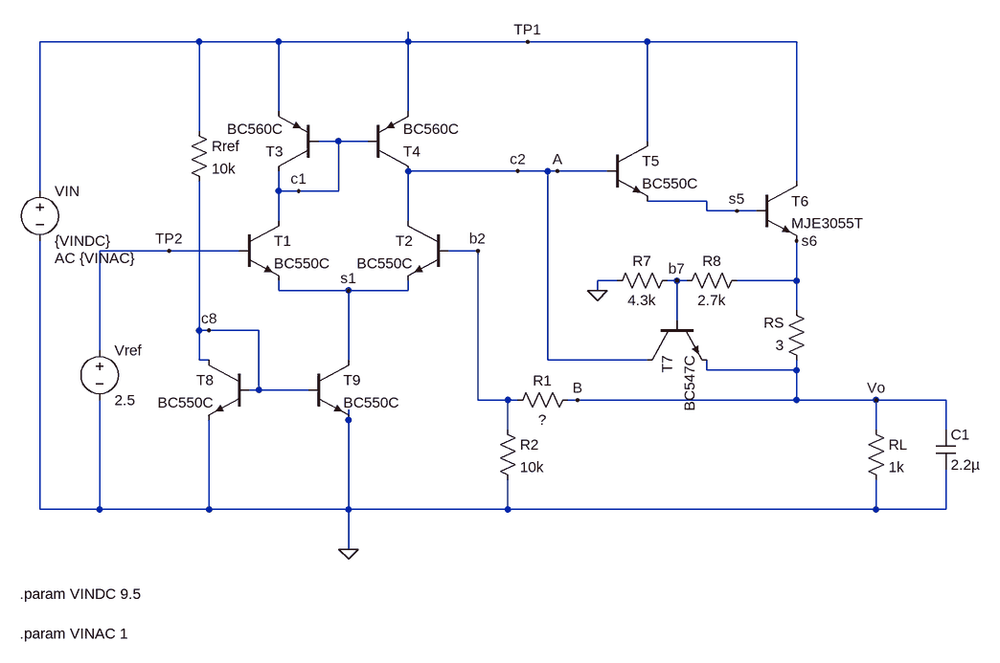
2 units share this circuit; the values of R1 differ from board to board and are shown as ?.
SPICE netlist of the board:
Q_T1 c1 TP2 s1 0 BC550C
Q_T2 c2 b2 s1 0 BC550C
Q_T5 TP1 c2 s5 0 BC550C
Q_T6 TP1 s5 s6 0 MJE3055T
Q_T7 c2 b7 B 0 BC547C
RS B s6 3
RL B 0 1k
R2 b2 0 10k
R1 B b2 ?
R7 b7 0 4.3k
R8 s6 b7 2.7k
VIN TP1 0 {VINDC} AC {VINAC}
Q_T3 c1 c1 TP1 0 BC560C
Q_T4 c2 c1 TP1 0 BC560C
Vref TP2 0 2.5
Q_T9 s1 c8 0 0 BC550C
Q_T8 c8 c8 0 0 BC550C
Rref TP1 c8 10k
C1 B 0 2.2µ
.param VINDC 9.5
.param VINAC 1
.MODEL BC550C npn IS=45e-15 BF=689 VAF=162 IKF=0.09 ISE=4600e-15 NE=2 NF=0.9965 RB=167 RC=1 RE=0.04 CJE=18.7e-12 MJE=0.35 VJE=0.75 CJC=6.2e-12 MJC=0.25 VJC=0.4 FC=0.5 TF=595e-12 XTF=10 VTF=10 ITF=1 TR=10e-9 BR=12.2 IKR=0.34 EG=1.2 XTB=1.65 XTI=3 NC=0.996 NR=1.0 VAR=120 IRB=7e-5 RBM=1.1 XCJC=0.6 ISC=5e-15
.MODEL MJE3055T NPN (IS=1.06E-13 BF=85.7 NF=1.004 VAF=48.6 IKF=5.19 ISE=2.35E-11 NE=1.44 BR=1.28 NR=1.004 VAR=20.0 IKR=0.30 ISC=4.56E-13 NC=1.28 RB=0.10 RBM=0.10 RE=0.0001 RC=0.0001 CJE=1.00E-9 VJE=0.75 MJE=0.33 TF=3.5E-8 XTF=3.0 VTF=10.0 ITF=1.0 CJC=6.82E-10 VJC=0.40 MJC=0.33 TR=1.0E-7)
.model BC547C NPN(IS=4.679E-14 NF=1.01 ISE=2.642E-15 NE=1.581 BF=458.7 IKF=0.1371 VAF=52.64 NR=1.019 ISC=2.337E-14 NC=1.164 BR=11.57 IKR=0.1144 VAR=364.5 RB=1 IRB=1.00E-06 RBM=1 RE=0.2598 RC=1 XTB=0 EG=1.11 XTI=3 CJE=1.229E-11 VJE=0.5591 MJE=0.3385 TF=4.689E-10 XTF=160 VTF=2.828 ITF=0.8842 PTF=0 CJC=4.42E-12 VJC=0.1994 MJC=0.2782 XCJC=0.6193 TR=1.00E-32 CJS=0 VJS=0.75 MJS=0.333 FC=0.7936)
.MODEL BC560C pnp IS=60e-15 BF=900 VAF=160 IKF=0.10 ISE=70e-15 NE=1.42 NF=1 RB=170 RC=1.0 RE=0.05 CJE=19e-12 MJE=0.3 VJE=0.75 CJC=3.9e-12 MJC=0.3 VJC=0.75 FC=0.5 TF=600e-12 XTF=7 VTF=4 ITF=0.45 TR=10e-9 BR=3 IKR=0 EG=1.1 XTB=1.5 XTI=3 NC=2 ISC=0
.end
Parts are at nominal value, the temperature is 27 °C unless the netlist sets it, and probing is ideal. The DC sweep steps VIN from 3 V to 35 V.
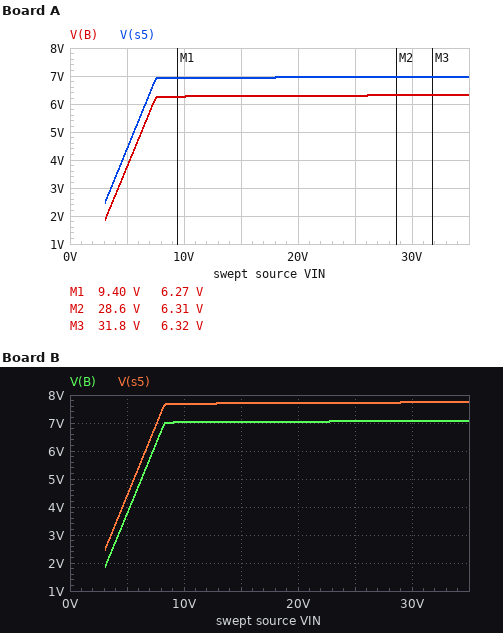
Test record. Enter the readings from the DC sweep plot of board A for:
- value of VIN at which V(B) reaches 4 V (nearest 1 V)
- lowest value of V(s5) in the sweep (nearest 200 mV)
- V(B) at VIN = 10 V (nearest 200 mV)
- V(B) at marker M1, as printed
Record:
5 V
2.4 V
6.2 V
6.27 V
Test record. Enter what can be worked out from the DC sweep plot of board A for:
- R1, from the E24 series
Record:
15 kΩ
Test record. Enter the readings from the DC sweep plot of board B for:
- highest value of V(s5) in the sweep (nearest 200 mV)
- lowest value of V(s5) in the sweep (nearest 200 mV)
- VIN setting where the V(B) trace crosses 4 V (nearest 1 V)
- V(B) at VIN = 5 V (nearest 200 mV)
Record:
7.8 V
2.4 V
5 V
3.8 V
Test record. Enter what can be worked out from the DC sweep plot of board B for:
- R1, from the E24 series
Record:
18 kΩ
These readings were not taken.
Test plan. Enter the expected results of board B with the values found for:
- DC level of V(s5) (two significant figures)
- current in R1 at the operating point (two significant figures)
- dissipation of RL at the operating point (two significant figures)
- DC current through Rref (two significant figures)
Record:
7.7 V
250 µA
49 mW
890 µA
